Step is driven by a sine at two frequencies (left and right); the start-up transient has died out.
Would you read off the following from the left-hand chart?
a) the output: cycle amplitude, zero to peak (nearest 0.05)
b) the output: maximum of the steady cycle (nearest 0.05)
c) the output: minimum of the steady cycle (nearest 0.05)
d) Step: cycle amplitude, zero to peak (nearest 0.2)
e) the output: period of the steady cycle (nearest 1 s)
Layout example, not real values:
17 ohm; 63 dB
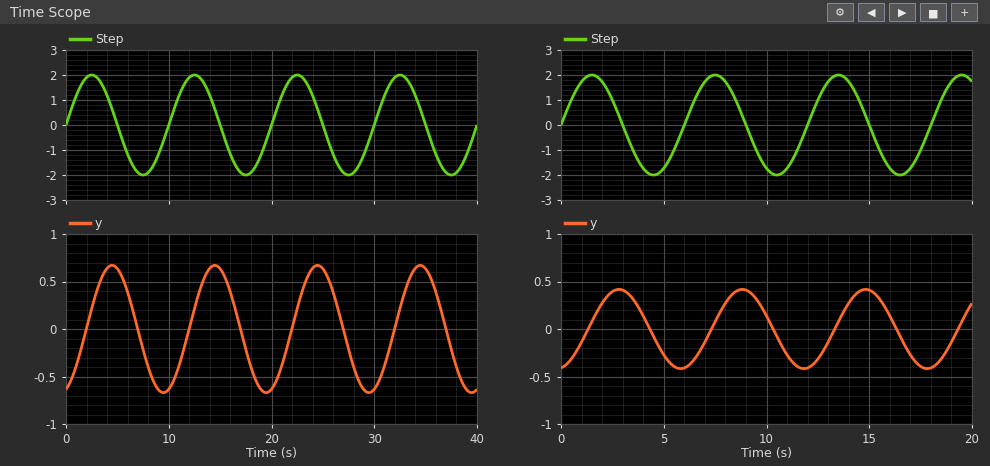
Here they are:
0.65; 0.65; -0.65; 2.0; 10 s
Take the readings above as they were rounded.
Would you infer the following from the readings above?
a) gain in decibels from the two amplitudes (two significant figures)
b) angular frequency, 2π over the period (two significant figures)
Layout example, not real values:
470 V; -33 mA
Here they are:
-9.8 dB; 0.63 rad/s
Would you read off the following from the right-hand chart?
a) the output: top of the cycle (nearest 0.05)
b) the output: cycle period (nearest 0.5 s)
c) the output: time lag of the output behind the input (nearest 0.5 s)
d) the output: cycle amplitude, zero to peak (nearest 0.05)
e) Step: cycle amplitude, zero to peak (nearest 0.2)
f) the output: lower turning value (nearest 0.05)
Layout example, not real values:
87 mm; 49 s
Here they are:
0.40; 6.0 s; 1.5 s; 0.40; 2.0; -0.40
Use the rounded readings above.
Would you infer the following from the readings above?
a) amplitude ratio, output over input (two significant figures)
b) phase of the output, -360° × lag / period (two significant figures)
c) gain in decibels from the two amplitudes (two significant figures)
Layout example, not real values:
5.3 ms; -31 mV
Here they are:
0.20; -90°; -14 dB
